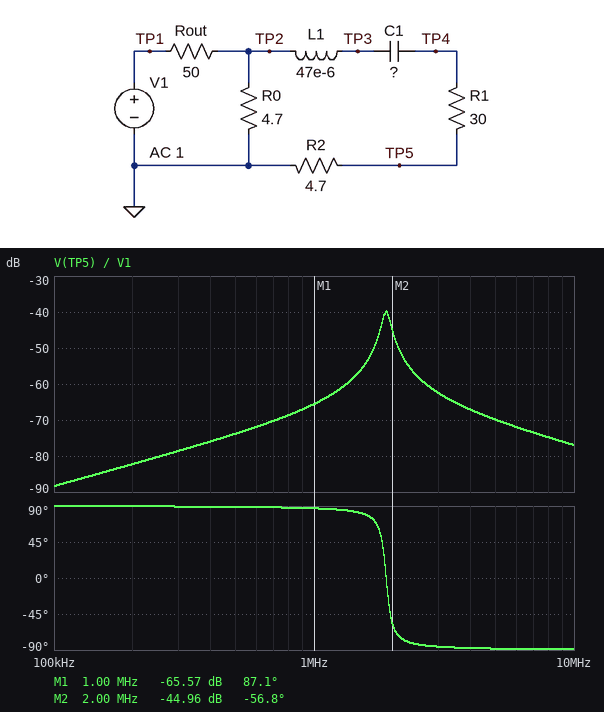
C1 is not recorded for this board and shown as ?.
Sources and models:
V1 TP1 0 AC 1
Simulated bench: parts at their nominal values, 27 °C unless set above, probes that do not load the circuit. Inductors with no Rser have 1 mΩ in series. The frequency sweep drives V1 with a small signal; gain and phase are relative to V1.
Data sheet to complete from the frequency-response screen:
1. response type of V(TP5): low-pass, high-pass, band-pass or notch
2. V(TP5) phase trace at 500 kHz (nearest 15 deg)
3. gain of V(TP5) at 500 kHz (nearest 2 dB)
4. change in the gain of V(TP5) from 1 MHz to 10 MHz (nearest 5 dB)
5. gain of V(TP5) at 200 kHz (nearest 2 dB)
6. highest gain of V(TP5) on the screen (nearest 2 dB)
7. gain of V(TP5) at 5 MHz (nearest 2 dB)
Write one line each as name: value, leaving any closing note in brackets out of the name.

response type of V(TP5): low-pass, high-pass, band-pass or notch: band-pass
V(TP5) phase trace at 500 kHz: 90 deg
gain of V(TP5) at 500 kHz: -74 dB
change in the gain of V(TP5) from 1 MHz to 10 MHz: -10 dB
gain of V(TP5) at 200 kHz: -82 dB
highest gain of V(TP5) on the screen: -40 dB
gain of V(TP5) at 5 MHz: -70 dB
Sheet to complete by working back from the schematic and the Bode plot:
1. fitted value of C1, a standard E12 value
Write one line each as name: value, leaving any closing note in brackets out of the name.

fitted value of C1, a standard E12 value: 150 pF
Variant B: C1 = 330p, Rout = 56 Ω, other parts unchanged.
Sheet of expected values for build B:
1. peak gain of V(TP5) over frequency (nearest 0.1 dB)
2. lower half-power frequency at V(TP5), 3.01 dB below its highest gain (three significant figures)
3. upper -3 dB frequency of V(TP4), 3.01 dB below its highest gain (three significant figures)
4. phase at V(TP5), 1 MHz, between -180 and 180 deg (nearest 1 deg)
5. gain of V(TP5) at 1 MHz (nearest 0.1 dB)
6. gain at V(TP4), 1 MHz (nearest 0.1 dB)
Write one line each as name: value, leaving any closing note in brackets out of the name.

peak gain of V(TP5) over frequency: -40.6 dB
lower half-power frequency at V(TP5), 3.01 dB below its highest gain: 1.21 MHz
upper -3 dB frequency of V(TP4), 3.01 dB below its highest gain: 1.35 MHz
phase at V(TP5), 1 MHz, between -180 and 180 deg: 78 deg
gain of V(TP5) at 1 MHz: -54.4 dB
gain at V(TP4), 1 MHz: -37.0 dB
